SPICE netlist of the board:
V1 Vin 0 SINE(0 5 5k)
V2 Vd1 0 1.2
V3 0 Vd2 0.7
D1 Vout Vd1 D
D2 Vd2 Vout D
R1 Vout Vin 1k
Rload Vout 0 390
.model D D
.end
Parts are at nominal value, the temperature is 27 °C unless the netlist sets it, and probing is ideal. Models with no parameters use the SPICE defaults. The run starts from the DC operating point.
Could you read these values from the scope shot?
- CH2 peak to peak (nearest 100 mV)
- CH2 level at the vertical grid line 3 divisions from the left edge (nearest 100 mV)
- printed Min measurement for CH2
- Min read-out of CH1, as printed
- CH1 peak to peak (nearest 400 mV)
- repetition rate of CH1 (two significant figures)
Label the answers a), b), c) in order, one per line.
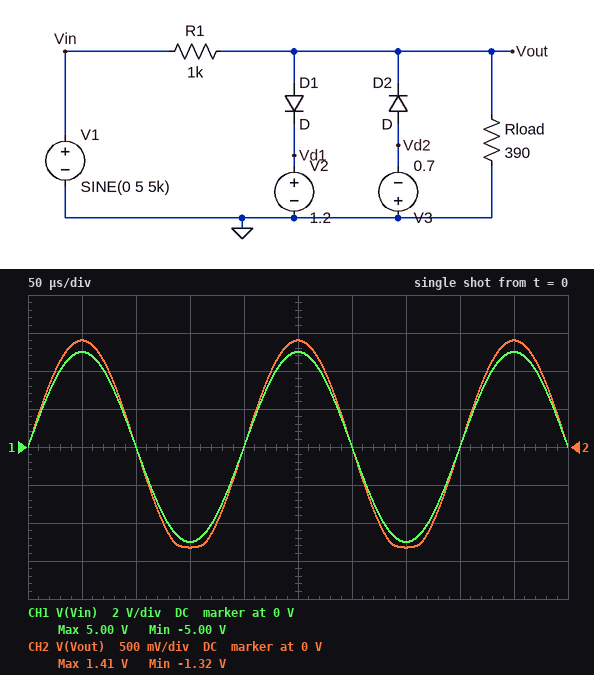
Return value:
a) 2.7 V
b) -1.3 V
c) -1.32 V
d) -5.00 V
e) 10.0 V
f) 5.0 kHz
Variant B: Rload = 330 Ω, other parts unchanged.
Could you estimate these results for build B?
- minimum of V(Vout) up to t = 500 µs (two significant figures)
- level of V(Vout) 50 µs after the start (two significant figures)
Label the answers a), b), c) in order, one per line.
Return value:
a) -1.2 V
b) 1.2 V
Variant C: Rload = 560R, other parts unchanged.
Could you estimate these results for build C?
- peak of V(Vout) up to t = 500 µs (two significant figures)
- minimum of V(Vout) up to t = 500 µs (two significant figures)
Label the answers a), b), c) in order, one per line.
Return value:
a) 1.8 V
b) -1.4 V
